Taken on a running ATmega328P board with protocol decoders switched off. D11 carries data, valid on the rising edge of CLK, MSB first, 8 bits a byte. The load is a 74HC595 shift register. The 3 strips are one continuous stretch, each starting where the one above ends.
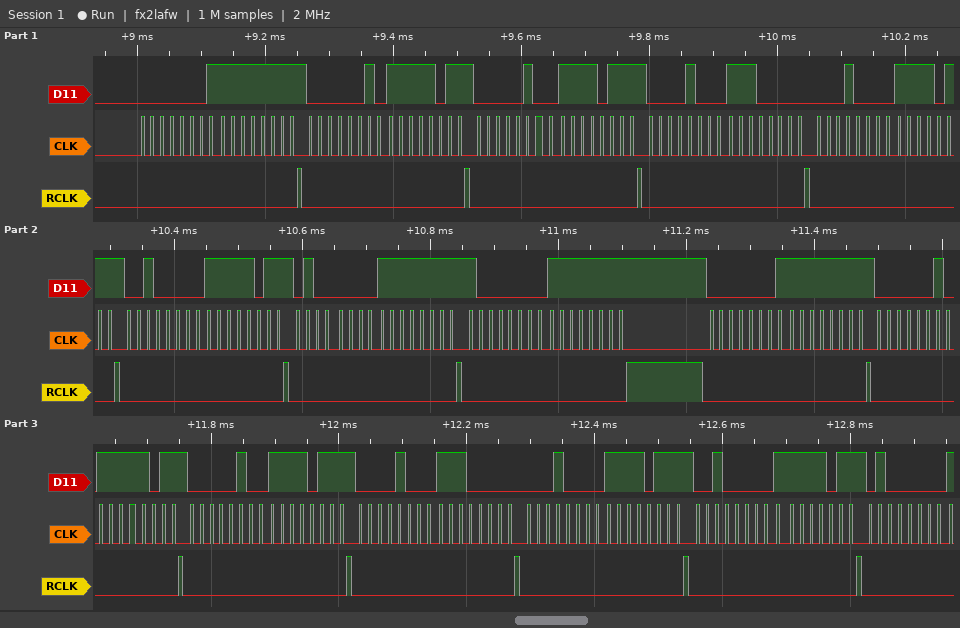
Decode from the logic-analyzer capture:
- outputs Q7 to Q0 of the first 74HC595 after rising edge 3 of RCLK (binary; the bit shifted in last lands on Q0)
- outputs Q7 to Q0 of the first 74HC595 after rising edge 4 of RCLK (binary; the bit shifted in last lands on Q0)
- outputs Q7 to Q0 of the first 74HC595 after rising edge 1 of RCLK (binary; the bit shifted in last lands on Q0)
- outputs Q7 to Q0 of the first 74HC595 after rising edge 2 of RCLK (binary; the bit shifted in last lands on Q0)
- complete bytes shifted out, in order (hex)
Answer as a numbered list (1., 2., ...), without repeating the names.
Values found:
1. 11110111
2. 11100000
3. 11111111
4. 11111011
5. 0x01 0xFF 0x02 0xFB 0x04 0xF7 0x08 0xE0 0x10 0xF7 0x20 0xFB 0x40 0xFF 0x80 0xFF 0x01 0xFF 0x02 0xFB 0x04 0xF7 0x08 0xE0 0x10 0xF7 0x20 0xFB 0x40
